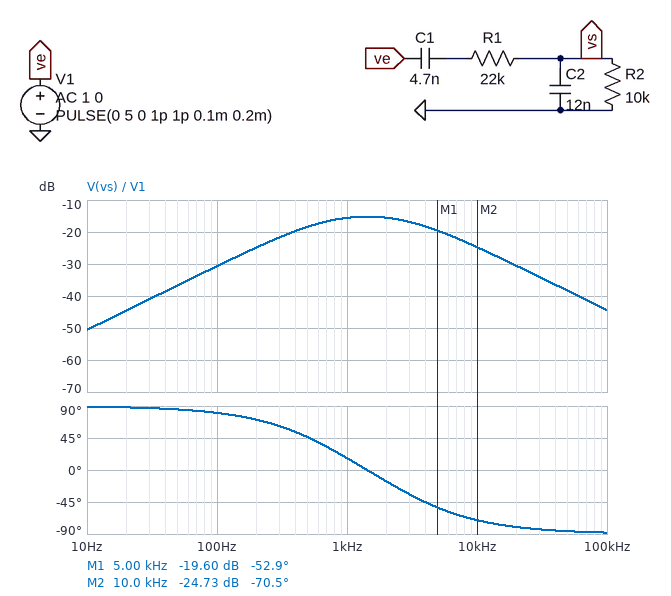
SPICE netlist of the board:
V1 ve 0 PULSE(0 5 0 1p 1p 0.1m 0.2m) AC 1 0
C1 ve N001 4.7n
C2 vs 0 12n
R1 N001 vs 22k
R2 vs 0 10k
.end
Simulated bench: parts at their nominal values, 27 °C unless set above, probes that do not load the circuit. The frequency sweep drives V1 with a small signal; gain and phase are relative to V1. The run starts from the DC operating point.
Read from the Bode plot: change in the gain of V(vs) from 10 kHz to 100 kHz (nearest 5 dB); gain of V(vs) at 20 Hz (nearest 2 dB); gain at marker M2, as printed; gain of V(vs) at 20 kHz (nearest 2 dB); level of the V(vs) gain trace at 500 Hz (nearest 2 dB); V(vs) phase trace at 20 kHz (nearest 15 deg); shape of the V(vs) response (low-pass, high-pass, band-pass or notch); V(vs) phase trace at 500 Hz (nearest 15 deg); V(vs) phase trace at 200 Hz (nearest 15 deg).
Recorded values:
-20 dB
-44 dB
-24.73 dB
-30 dB
-18 dB
-75 deg
band-pass
45 deg
75 deg
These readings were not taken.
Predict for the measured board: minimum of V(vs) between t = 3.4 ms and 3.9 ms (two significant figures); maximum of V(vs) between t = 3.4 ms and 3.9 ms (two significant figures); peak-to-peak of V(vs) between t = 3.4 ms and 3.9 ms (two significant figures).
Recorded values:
-350 mV
350 mV
710 mV
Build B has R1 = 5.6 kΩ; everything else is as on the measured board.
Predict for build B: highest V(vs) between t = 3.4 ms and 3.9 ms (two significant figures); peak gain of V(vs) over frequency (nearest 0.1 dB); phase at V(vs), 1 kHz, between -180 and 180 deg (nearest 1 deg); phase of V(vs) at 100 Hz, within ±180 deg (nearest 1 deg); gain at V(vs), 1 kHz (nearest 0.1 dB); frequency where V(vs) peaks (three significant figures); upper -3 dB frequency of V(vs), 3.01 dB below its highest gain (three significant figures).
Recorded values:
630 mV
-12.3 dB
36 deg
83 deg
-14.1 dB
2.83 kHz
10.5 kHz
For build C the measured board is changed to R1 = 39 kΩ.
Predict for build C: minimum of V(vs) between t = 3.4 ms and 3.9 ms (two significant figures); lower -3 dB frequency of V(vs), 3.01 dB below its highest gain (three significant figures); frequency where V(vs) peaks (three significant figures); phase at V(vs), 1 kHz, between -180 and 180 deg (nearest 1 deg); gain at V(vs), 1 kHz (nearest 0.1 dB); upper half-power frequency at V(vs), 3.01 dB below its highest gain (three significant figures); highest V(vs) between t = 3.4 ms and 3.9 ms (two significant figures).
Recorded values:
-230 mV
393 Hz
1.07 kHz
3 deg
-17.5 dB
2.93 kHz
230 mV
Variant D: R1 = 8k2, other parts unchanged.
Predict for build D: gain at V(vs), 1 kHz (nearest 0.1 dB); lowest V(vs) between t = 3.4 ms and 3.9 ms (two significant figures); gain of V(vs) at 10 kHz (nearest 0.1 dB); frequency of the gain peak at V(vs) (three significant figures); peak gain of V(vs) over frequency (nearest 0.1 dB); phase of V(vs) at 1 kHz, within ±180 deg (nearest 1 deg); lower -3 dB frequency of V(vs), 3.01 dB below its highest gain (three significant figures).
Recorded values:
-14.3 dB
-560 mV
-17.3 dB
2.34 kHz
-12.8 dB
32 deg
704 Hz
